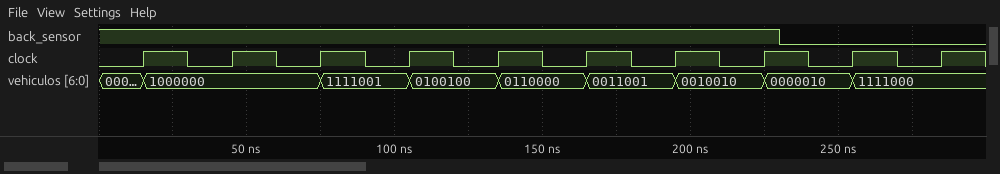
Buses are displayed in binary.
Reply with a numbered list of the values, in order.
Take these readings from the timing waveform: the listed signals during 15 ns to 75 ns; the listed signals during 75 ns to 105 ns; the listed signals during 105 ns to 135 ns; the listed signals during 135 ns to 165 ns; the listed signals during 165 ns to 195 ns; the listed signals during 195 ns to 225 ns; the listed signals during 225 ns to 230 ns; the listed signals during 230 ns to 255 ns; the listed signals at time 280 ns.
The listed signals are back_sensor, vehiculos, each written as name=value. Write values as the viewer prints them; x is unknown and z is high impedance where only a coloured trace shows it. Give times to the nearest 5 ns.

1. back_sensor=1, vehiculos=1000000
2. back_sensor=1, vehiculos=1111001
3. back_sensor=1, vehiculos=0100100
4. back_sensor=1, vehiculos=0110000
5. back_sensor=1, vehiculos=0011001
6. back_sensor=1, vehiculos=0010010
7. back_sensor=1, vehiculos=0000010
8. back_sensor=0, vehiculos=0000010
9. back_sensor=0, vehiculos=1111000
